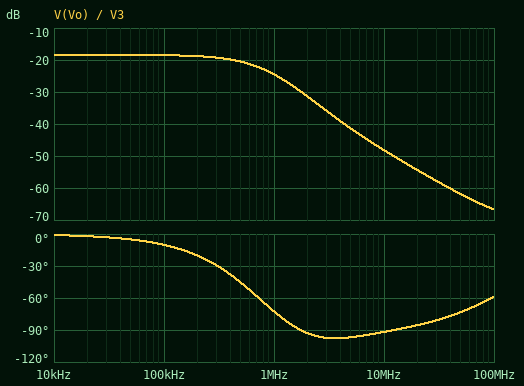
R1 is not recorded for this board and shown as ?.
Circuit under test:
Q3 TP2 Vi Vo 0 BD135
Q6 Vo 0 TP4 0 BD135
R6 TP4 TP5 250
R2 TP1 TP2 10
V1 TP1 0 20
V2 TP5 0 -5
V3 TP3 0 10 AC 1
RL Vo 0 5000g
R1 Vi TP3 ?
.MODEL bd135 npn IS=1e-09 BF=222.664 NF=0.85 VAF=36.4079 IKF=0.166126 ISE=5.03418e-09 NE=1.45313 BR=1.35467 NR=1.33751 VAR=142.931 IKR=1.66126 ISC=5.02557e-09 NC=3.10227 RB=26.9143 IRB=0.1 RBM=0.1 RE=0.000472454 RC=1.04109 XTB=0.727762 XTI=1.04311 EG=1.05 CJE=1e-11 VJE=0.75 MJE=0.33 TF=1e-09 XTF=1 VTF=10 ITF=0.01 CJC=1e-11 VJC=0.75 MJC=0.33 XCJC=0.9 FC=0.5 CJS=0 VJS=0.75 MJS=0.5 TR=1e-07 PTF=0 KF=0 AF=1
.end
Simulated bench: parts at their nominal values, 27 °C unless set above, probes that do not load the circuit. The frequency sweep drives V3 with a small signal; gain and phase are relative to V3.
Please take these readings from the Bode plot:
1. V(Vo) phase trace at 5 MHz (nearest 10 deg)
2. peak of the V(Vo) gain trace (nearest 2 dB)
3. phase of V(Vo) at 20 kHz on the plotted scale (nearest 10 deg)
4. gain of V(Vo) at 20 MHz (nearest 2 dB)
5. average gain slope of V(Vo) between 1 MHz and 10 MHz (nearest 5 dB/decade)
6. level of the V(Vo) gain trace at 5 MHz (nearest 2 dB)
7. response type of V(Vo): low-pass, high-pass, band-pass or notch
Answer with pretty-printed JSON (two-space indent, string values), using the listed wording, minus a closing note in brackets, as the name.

{
  "V(Vo) phase trace at 5 MHz": "-100 deg",
  "peak of the V(Vo) gain trace": "-18 dB",
  "phase of V(Vo) at 20 kHz on the plotted scale": "0 deg",
  "gain of V(Vo) at 20 MHz": "-54 dB",
  "average gain slope of V(Vo) between 1 MHz and 10 MHz": "-25 dB/decade",
  "level of the V(Vo) gain trace at 5 MHz": "-42 dB",
  "response type of V(Vo): low-pass, high-pass, band-pass or notch": "low-pass"
}
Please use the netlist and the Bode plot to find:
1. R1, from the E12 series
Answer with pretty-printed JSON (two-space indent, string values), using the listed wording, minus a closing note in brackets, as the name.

{
  "R1, from the E12 series": "82 kΩ"
}
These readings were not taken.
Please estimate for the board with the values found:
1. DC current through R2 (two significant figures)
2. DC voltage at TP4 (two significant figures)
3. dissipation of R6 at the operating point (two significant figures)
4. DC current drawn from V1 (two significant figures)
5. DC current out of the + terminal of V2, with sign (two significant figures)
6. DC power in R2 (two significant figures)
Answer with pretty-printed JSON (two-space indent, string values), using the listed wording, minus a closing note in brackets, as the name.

{
  "DC current through R2": "17 mA",
  "DC voltage at TP4": "-400 mV",
  "dissipation of R6 at the operating point": "85 mW",
  "DC current drawn from V1": "17 mA",
  "DC current out of the + terminal of V2, with sign": "-18 mA",
  "DC power in R2": "3.0 mW"
}
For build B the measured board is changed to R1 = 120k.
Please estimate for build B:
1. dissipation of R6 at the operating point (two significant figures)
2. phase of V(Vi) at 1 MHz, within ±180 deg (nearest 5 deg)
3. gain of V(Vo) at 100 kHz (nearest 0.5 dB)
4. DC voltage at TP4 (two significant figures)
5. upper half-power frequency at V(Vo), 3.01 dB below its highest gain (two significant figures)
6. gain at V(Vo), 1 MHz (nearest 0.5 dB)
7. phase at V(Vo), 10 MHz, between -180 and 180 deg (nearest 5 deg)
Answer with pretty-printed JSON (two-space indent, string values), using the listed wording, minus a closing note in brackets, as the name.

{
  "dissipation of R6 at the operating point": "80 mW",
  "phase of V(Vi) at 1 MHz, within ±180 deg": "-55 deg",
  "gain of V(Vo) at 100 kHz": "-29.0 dB",
  "DC voltage at TP4": "-540 mV",
  "upper half-power frequency at V(Vo), 3.01 dB below its highest gain": "730 kHz",
  "gain at V(Vo), 1 MHz": "-33.5 dB",
  "phase at V(Vo), 10 MHz, between -180 and 180 deg": "-85 deg"
}
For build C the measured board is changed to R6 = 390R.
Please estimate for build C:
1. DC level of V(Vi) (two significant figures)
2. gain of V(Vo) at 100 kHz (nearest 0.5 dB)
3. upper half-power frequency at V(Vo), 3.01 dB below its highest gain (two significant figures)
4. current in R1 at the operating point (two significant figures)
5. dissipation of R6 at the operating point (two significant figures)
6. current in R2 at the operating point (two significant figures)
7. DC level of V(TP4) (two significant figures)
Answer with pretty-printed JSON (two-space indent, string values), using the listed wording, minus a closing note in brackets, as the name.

{
  "DC level of V(Vi)": "2.4 V",
  "gain of V(Vo) at 100 kHz": "-1.0 dB",
  "upper half-power frequency at V(Vo), 3.01 dB below its highest gain": "600 kHz",
  "current in R1 at the operating point": "93 µA",
  "dissipation of R6 at the operating point": "55 mW",
  "current in R2 at the operating point": "12 mA",
  "DC level of V(TP4)": "-360 mV"
}
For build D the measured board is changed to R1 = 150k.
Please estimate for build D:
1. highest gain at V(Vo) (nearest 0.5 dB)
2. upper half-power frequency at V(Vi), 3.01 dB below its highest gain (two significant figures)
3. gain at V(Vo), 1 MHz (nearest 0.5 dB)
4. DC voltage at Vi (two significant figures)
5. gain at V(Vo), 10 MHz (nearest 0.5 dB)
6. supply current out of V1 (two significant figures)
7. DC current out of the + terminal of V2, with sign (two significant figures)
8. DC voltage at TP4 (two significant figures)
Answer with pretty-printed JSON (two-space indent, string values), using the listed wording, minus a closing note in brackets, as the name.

{
  "highest gain at V(Vo)": "-31.5 dB",
  "upper half-power frequency at V(Vi), 3.01 dB below its highest gain": "780 kHz",
  "gain at V(Vo), 1 MHz": "-36.0 dB",
  "DC voltage at Vi": "-420 mV",
  "gain at V(Vo), 10 MHz": "-54.5 dB",
  "supply current out of V1": "8.4 mA",
  "DC current out of the + terminal of V2, with sign": "-18 mA",
  "DC voltage at TP4": "-590 mV"
}
